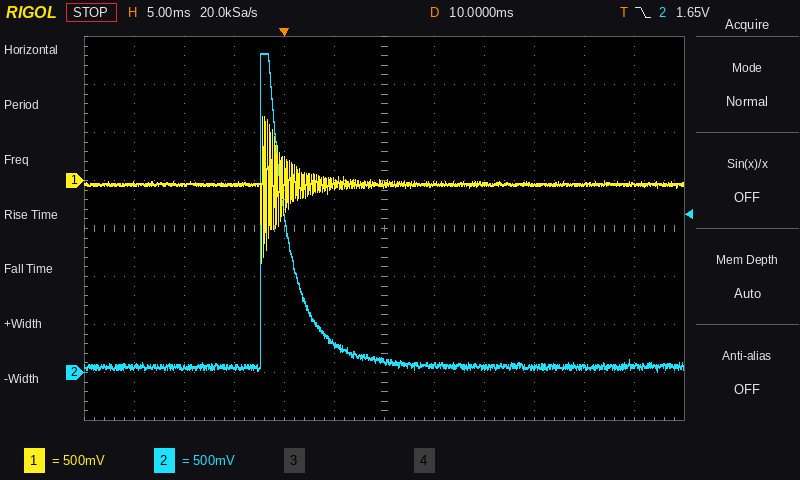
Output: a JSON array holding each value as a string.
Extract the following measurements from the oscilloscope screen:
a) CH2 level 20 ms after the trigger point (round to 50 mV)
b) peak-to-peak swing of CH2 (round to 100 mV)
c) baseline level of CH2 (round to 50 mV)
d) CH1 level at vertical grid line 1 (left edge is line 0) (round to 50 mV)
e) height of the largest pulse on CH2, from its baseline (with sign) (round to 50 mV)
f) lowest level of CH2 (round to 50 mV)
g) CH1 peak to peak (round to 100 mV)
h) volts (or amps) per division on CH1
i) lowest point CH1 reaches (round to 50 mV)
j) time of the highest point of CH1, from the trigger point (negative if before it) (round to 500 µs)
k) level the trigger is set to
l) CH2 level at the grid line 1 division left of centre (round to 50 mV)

["50 mV", "3.30 V", "50 mV", "-50 mV", "+3.25 V", "0 mV", "1.50 V", "500 mV", "-850 mV", "-2.0 ms", "1.65 V", "300 mV"]
